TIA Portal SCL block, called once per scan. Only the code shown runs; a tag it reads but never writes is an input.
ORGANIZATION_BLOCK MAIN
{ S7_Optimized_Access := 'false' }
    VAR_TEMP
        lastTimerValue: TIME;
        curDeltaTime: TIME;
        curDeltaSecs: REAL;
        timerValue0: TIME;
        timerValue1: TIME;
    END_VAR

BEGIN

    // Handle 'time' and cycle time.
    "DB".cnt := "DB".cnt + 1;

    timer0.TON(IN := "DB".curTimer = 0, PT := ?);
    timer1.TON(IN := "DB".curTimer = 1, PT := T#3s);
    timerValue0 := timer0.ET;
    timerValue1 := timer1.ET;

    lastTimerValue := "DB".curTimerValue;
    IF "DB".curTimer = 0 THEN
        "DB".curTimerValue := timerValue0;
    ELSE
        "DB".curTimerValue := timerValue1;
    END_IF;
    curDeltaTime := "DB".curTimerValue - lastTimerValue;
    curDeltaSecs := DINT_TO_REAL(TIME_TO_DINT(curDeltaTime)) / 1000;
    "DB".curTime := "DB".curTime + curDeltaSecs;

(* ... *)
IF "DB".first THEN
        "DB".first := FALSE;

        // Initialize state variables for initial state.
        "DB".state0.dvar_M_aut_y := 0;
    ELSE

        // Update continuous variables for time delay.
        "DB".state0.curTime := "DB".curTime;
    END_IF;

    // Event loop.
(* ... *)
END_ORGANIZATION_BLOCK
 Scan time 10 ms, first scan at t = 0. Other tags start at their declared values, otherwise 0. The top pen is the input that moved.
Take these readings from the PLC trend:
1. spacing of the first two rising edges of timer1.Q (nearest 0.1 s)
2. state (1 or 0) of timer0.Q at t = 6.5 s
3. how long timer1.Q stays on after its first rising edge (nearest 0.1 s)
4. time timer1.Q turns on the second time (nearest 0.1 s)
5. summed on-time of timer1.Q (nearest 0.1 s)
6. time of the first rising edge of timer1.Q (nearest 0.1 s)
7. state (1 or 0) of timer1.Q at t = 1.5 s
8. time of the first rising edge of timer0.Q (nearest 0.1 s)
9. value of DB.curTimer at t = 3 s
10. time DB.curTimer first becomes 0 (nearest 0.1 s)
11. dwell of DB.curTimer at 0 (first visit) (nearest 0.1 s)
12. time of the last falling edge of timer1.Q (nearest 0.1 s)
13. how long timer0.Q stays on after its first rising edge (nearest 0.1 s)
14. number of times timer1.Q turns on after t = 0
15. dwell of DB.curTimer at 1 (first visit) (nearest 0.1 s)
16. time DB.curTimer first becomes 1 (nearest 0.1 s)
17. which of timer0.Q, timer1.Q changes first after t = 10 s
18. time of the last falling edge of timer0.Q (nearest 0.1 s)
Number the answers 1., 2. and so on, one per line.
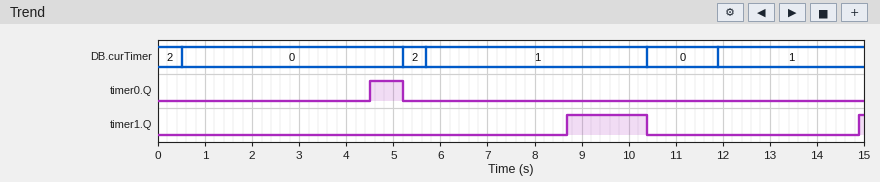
1. 6.2 s
2. 0
3. 1.7 s
4. 14.9 s
5. 1.8 s
6. 8.7 s
7. 0
8. 4.5 s
9. 0
10. 0.5 s
11. 4.7 s
12. 10.4 s
13. 0.7 s
14. 2
15. 4.7 s
16. 5.7 s
17. timer1.Q
18. 5.2 s
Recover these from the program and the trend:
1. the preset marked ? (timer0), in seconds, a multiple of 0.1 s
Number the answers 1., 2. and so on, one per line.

1. 4.0 s
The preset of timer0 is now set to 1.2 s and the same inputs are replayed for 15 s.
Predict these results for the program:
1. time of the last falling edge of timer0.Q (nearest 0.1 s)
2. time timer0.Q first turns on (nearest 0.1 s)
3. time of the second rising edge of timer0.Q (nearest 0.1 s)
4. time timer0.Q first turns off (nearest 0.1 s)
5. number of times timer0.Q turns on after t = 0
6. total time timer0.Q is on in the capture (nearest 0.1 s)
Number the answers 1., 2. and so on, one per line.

1. 11.9 s
2. 1.7 s
3. 11.6 s
4. 5.2 s
5. 2
6. 3.8 s
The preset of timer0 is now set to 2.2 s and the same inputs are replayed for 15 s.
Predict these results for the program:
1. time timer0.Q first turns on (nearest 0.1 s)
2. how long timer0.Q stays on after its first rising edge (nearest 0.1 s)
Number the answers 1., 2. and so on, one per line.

1. 2.7 s
2. 2.5 s
